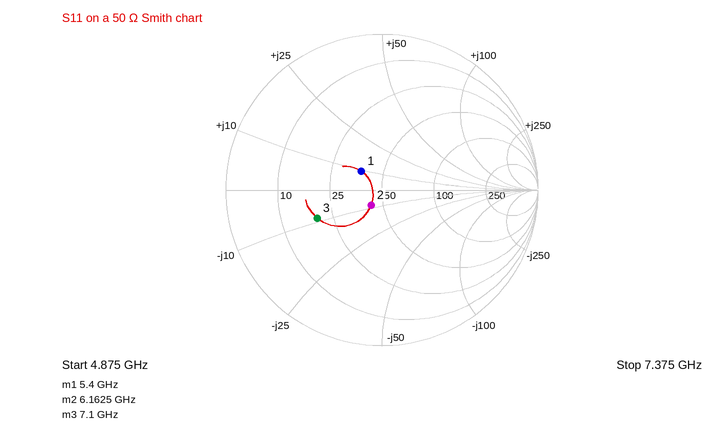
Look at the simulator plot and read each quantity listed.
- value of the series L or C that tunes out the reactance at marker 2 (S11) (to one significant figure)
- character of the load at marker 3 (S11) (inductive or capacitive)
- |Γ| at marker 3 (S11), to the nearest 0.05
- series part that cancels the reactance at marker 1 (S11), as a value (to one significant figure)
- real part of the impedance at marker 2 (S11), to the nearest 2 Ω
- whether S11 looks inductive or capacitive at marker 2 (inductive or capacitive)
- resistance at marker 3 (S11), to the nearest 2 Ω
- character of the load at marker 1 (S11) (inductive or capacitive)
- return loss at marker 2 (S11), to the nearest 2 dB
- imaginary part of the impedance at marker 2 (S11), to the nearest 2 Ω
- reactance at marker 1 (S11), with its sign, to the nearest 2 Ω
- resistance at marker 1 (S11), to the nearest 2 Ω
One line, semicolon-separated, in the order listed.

200 pH; capacitive; 0.45; 3 pF; 42 Ω; capacitive; 20 Ω; inductive; 18 dB; -8 Ω; +10 Ω; 38 Ω
